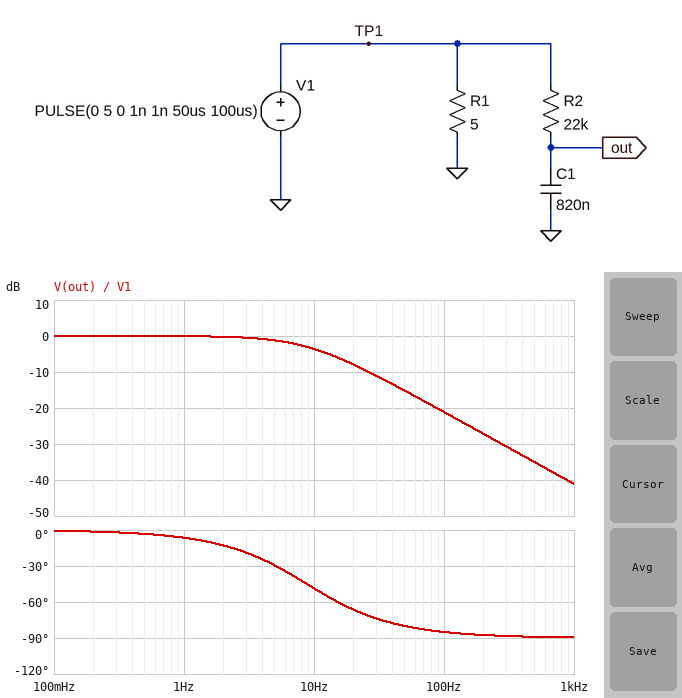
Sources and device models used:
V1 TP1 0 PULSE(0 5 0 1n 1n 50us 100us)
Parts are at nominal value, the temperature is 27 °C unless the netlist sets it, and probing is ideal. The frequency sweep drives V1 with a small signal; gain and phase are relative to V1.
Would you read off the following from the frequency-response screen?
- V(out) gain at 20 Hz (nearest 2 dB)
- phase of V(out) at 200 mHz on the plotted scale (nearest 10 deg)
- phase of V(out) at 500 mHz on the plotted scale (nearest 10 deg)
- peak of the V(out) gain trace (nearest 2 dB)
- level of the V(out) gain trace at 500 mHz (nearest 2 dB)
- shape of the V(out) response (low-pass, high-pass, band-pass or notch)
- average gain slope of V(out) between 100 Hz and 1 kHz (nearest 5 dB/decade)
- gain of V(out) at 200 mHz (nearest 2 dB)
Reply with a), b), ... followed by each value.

a) -8 dB
b) 0 deg
c) 0 deg
d) 0 dB
e) 0 dB
f) low-pass
g) -20 dB/decade
h) 0 dB
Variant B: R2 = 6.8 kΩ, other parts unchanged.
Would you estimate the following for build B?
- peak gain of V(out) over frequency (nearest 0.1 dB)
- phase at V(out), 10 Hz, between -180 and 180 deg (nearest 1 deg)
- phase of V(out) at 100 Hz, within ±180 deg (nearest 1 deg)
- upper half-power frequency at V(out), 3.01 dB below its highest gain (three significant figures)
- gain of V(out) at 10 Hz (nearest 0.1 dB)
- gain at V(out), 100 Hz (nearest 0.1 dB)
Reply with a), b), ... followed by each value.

a) 0 dB
b) -19 deg
c) -74 deg
d) 28.5 Hz
e) -0.5 dB
f) -11.2 dB
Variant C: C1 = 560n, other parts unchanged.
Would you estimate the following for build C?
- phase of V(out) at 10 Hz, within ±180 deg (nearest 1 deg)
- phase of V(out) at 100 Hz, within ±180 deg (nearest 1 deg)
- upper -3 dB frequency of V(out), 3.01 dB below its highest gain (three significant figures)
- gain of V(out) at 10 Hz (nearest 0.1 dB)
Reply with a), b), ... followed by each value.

a) -38 deg
b) -83 deg
c) 12.9 Hz
d) -2.0 dB
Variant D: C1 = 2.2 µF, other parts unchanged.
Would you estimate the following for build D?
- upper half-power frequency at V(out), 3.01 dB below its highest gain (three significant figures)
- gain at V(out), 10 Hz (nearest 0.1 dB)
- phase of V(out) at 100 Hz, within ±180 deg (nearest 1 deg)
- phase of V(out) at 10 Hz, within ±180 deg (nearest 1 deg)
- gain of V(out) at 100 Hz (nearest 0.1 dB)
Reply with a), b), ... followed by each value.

a) 3.29 Hz
b) -10.1 dB
c) -88 deg
d) -72 deg
e) -29.7 dB
